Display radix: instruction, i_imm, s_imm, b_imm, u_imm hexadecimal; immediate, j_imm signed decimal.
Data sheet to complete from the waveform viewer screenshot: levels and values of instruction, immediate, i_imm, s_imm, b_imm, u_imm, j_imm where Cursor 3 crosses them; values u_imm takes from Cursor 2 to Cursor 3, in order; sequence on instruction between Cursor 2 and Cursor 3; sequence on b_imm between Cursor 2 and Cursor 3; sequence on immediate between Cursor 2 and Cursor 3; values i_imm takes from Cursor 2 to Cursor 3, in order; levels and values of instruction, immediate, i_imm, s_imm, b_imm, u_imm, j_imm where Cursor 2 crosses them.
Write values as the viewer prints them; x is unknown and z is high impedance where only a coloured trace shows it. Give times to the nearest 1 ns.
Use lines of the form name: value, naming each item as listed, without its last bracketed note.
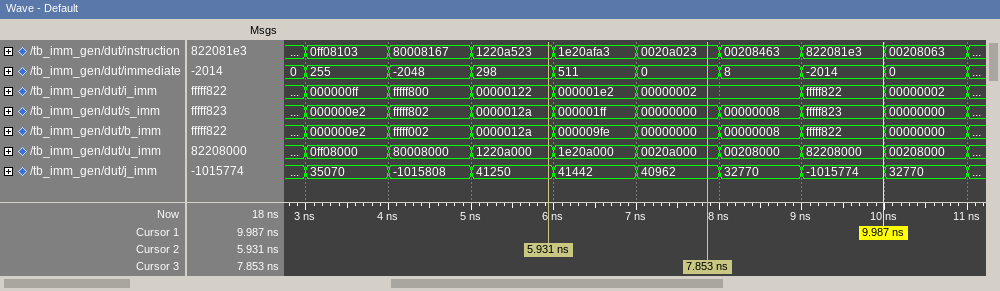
levels and values of instruction, immediate, i_imm, s_imm, b_imm, u_imm, j_imm where Cursor 3 crosses them: instruction=0020a023, immediate=0, i_imm=00000002, s_imm=00000000, b_imm=00000000, u_imm=0020a000, j_imm=40962
values u_imm takes from Cursor 2 to Cursor 3, in order: 1220a000, 1e20a000, 0020a000
sequence on instruction between Cursor 2 and Cursor 3: 1220a523, 1e20afa3, 0020a023
sequence on b_imm between Cursor 2 and Cursor 3: 0000012a, 000009fe, 00000000
sequence on immediate between Cursor 2 and Cursor 3: 298, 511, 0
values i_imm takes from Cursor 2 to Cursor 3, in order: 00000122, 000001e2, 00000002
levels and values of instruction, immediate, i_imm, s_imm, b_imm, u_imm, j_imm where Cursor 2 crosses them: instruction=1220a523, immediate=298, i_imm=00000122, s_imm=0000012a, b_imm=0000012a, u_imm=1220a000, j_imm=41250
